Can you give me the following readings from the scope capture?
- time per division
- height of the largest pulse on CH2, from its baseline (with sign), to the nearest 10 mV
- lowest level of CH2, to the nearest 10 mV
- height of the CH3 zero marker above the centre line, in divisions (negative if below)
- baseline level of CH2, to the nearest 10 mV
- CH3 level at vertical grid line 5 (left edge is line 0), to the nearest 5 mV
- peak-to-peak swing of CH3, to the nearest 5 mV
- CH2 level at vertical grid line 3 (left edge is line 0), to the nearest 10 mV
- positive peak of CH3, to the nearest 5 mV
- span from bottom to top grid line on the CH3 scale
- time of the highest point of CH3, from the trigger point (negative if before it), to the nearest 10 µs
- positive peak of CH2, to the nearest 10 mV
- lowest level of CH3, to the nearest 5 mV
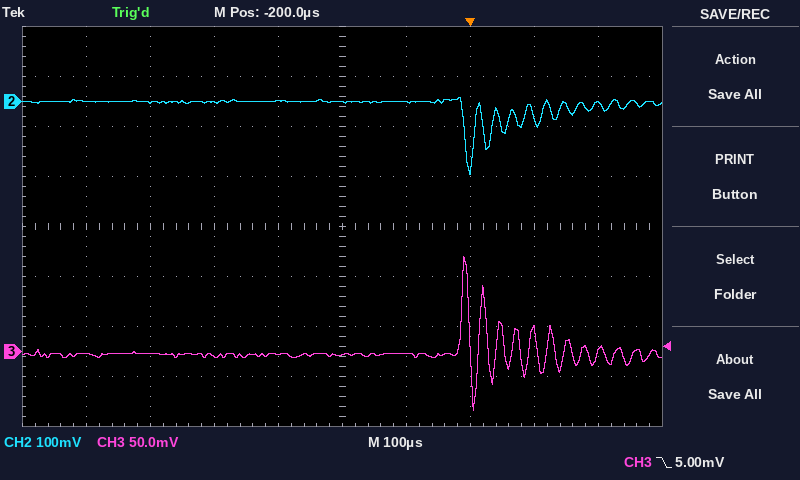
100 µs
-150 mV
-150 mV
-2.5 div
0 mV
-5 mV
155 mV
0 mV
95 mV
400 mV
-10 µs
10 mV
-60 mV
